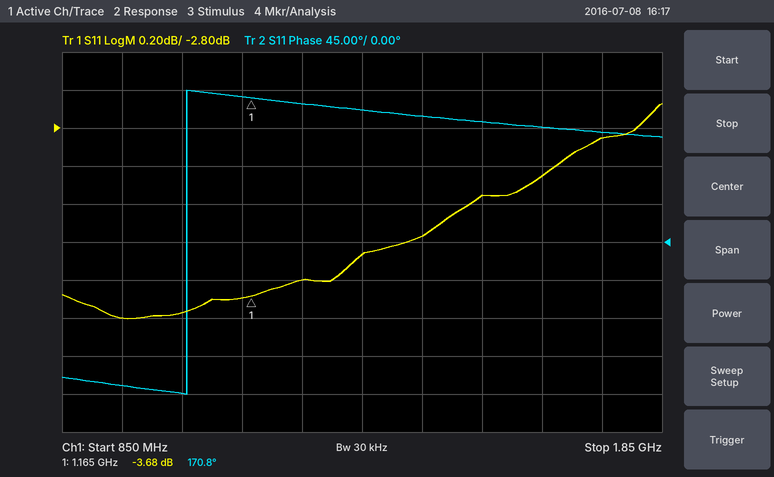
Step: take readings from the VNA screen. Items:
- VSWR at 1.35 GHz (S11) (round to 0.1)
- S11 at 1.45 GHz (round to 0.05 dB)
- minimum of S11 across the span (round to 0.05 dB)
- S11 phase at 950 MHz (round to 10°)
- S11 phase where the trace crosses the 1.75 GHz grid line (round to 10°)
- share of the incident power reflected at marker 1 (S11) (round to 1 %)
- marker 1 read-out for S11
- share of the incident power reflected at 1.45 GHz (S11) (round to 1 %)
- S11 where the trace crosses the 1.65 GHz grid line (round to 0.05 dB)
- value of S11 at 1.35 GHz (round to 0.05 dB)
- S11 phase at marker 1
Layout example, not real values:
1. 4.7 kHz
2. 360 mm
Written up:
1. 5.1
2. -3.35 dB
3. -3.80 dB
4. -170°
5. 130°
6. 43 %
7. -3.68 dB
8. 46 %
9. -3.05 dB
10. -3.45 dB
11. 170.8°
